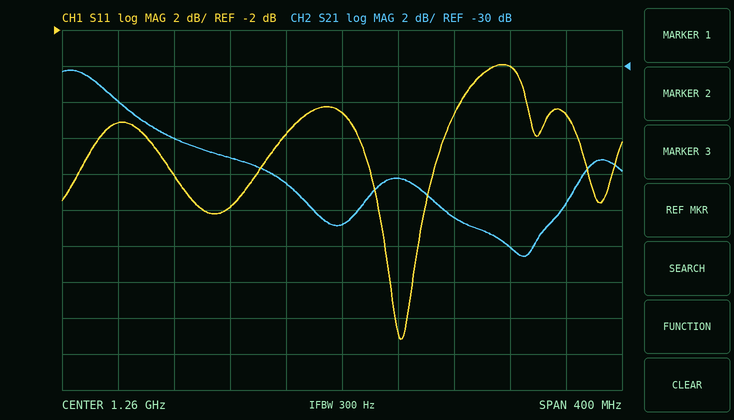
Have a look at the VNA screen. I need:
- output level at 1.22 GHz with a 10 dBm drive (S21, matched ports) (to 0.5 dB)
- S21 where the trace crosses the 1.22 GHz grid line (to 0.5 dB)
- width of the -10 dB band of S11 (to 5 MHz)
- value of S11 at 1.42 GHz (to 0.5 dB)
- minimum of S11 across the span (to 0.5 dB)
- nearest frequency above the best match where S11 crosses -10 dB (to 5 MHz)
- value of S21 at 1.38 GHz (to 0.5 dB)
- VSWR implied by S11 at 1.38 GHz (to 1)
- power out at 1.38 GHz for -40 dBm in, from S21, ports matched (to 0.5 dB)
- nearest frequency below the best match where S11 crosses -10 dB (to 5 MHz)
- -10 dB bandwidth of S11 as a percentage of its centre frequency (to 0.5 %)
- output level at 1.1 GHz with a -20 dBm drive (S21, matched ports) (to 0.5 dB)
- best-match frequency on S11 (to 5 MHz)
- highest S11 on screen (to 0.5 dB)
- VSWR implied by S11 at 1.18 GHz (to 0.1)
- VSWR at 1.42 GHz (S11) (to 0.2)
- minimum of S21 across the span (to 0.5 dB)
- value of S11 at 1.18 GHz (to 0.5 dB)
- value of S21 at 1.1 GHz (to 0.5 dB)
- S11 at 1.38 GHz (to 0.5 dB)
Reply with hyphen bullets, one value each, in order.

- -26.5 dBm
- -36.5 dB
- 45 MHz
- -6.5 dB
- -19.0 dB
- 1.325 GHz
- -40.0 dB
- 4
- -80.0 dBm
- 1.280 GHz
- 3.5 %
- -52.0 dBm
- 1.300 GHz
- -4.0 dB
- 1.7
- 2.8
- -40.5 dB
- -12.0 dB
- -32.0 dB
- -4.0 dB
